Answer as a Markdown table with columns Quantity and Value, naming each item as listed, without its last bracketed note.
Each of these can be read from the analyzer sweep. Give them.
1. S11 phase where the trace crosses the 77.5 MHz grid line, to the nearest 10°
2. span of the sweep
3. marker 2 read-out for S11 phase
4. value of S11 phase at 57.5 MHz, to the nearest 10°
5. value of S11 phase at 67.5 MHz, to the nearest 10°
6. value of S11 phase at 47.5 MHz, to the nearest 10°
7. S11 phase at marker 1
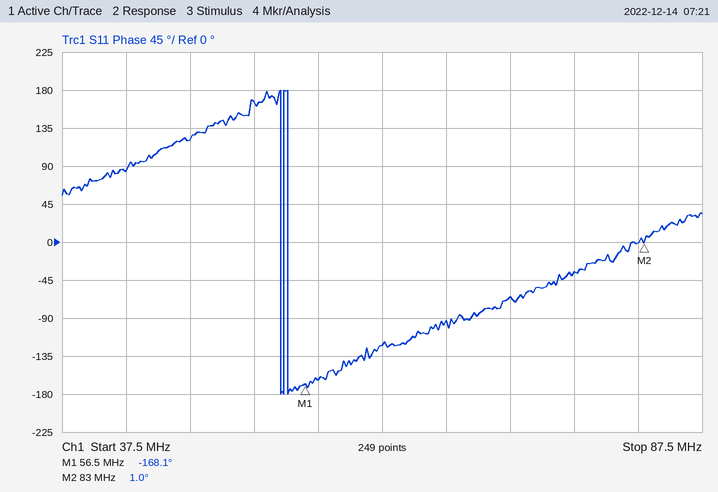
| Quantity | Value |
|---|---|
| S11 phase where the trace crosses the 77.5 MHz grid line, to the nearest 10° | -40° |
| span of the sweep | 50 MHz |
| marker 2 read-out for S11 phase | 1.0° |
| value of S11 phase at 57.5 MHz, to the nearest 10° | -160° |
| value of S11 phase at 67.5 MHz, to the nearest 10° | -90° |
| value of S11 phase at 47.5 MHz, to the nearest 10° | 120° |
| S11 phase at marker 1 | -168.1° |
